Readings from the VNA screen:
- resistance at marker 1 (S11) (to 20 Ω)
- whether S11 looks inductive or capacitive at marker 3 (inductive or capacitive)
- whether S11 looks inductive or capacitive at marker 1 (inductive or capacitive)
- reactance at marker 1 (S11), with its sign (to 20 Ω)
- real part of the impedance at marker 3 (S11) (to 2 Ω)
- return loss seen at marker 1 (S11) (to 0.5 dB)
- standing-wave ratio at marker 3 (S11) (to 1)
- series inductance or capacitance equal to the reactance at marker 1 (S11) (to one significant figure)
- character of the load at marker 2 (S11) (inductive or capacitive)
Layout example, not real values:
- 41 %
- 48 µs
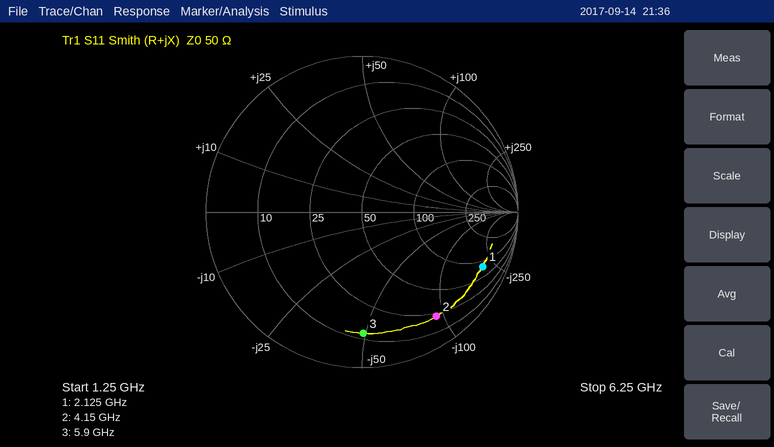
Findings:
- 80 Ω
- capacitive
- capacitive
- -200 Ω
- 12 Ω
- 1.5 dB
- 8
- 400 fF
- capacitive
